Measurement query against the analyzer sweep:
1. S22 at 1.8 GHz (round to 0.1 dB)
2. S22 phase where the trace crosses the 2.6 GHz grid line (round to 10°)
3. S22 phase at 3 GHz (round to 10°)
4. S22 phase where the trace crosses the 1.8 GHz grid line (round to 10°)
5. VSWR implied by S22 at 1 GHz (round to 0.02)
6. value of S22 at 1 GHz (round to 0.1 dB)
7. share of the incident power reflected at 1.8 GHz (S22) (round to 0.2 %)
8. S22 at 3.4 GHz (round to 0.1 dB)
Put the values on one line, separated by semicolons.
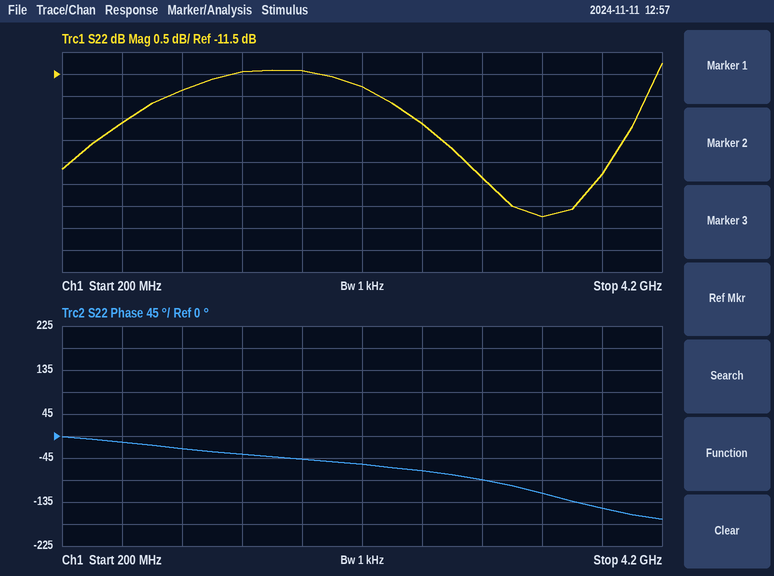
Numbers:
-11.4 dB; -70°; -90°; -50°; 1.68; -11.9 dB; 7.2 %; -14.7 dB
